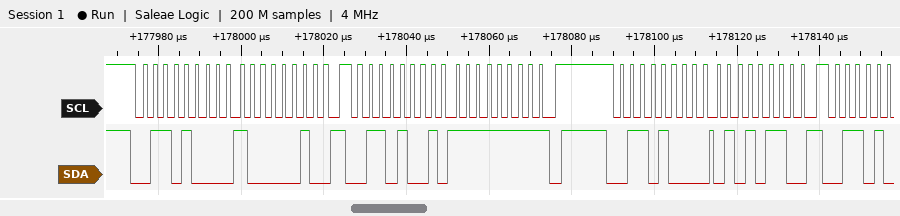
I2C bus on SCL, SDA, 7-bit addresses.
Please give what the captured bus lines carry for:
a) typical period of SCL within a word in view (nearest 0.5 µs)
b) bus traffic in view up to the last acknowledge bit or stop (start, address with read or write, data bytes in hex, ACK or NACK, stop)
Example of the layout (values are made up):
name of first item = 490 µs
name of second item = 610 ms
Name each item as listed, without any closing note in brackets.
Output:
typical period of SCL within a word in view = 2.5 µs
bus traffic in view up to the last acknowledge bit or stop = start, address 34 write ACK, 82 ACK, repeated start, address 34 read ACK, FF NACK, stop, start, address 34 write ACK, 56 ACK
